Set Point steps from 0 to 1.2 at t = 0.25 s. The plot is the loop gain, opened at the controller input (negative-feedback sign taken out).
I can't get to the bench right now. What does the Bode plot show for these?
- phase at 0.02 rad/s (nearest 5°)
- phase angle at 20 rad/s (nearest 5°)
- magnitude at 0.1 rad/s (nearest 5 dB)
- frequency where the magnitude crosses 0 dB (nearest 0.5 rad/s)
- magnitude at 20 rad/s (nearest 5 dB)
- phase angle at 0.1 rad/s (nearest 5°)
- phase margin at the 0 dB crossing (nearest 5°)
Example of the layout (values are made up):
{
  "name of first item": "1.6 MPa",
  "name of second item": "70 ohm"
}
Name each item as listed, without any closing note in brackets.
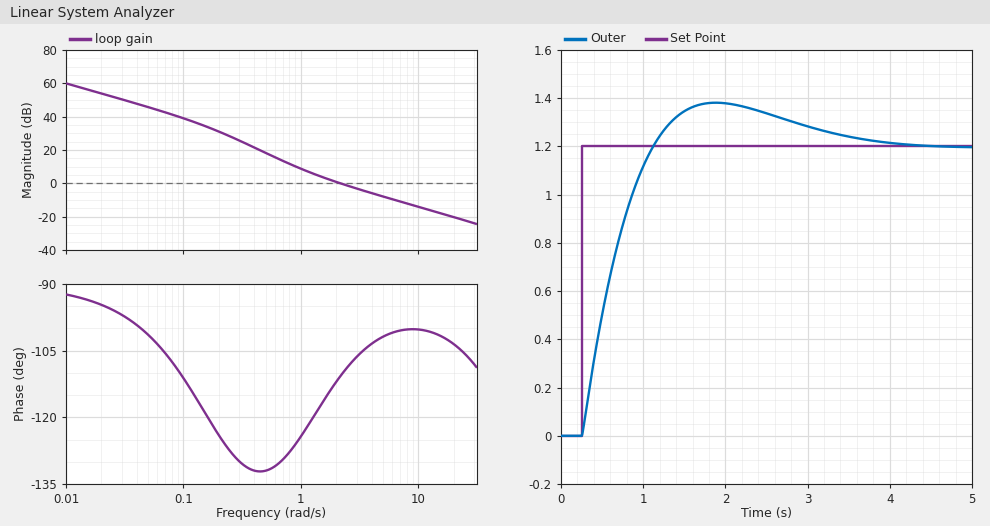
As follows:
{
  "phase at 0.02 rad/s": "-95°",
  "phase angle at 20 rad/s": "-105°",
  "magnitude at 0.1 rad/s": "40 dB",
  "frequency where the magnitude crosses 0 dB": "2.0 rad/s",
  "magnitude at 20 rad/s": "-20 dB",
  "phase angle at 0.1 rad/s": "-110°",
  "phase margin at the 0 dB crossing": "70°"
}
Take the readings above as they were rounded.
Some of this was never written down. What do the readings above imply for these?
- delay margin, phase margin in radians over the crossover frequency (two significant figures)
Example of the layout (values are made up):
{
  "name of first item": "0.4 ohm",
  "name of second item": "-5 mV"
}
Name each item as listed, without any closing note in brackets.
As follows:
{
  "delay margin, phase margin in radians over the crossover frequency": "0.61 s"
}
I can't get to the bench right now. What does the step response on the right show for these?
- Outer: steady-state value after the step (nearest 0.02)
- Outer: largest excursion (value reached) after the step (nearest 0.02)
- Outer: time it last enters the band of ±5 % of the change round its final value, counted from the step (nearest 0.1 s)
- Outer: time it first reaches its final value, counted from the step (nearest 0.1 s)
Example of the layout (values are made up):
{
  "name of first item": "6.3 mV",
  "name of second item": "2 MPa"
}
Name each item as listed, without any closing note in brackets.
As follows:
{
  "Outer: steady-state value after the step": "1.20",
  "Outer: largest excursion (value reached) after the step": "1.38",
  "Outer: time it last enters the band of ±5 % of the change round its final value, counted from the step": "3.0 s",
  "Outer: time it first reaches its final value, counted from the step": "0.9 s"
}
